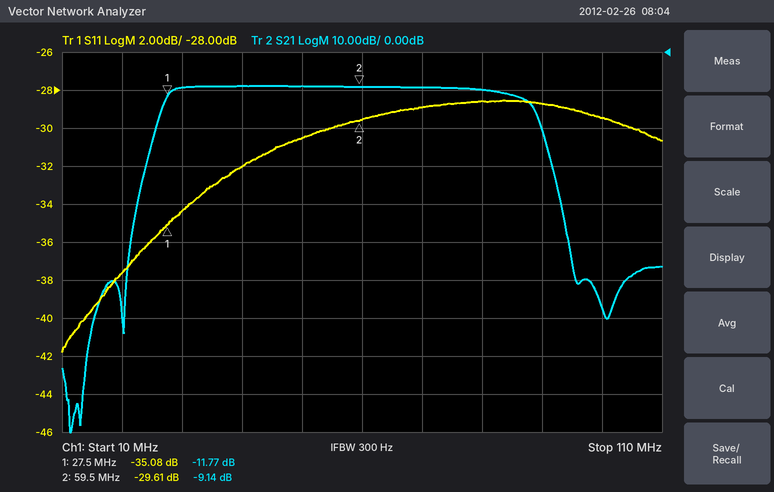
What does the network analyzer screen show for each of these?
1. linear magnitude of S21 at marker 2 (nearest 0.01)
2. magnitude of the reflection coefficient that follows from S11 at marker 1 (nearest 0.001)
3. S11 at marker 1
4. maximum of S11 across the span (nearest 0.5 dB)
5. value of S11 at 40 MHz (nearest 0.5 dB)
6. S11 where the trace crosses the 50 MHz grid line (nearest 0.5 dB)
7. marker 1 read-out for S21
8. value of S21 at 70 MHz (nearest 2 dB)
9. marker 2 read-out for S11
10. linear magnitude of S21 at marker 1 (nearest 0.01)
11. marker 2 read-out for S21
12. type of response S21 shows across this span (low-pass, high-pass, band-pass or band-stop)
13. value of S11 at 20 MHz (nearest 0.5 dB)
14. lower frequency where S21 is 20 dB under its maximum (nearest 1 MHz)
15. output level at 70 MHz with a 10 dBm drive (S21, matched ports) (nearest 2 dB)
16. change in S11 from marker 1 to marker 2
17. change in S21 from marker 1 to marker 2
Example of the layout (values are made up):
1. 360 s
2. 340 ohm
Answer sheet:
1. 0.35
2. 0.018
3. -35.08 dB
4. -28.5 dB
5. -32.0 dB
6. -30.5 dB
7. -11.77 dB
8. -10 dB
9. -29.61 dB
10. 0.26
11. -9.14 dB
12. band-pass
13. -37.5 dB
14. 24 MHz
15. 0 dBm
16. 5.47 dB
17. 2.63 dB
